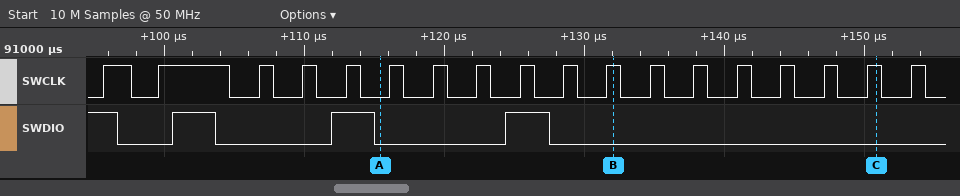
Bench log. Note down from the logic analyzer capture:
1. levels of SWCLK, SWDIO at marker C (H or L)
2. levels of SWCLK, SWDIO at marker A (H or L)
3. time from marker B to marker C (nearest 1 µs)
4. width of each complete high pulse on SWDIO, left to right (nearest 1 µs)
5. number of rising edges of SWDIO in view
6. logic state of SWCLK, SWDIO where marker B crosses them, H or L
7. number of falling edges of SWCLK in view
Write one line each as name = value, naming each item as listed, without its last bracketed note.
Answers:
levels of SWCLK, SWDIO at marker C = SWCLK=H, SWDIO=L
levels of SWCLK, SWDIO at marker A = SWCLK=L, SWDIO=L
time from marker B to marker C = 19 µs
width of each complete high pulse on SWDIO, left to right = 3 µs, 3 µs, 3 µs
number of rising edges of SWDIO in view = 3
logic state of SWCLK, SWDIO where marker B crosses them, H or L = SWCLK=H, SWDIO=L
number of falling edges of SWCLK in view = 18
